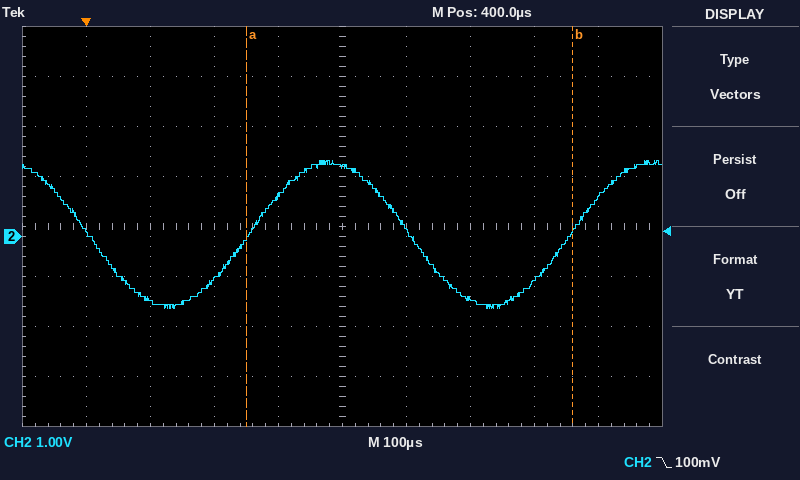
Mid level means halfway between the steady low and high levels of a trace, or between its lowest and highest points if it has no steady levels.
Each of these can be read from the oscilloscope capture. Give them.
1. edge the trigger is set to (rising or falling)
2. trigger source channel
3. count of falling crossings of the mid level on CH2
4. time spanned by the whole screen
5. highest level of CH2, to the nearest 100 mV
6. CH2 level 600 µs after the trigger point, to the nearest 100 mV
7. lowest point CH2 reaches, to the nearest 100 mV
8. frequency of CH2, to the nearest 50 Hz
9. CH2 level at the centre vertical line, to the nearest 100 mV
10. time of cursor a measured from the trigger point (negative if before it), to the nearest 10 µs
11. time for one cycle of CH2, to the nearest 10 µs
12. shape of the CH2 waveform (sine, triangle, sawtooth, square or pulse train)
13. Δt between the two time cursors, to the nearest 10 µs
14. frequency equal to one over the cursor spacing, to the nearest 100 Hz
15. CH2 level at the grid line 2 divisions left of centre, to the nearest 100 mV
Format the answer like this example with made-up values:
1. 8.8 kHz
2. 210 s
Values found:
1. falling
2. CH2
3. 2
4. 1 ms
5. 1.5 V
6. -1.2 V
7. -1.4 V
8. 2.00 kHz
9. 1.4 V
10. +250 µs
11. 500 µs
12. sine
13. 510 µs
14. 2.0 kHz
15. -900 mV
